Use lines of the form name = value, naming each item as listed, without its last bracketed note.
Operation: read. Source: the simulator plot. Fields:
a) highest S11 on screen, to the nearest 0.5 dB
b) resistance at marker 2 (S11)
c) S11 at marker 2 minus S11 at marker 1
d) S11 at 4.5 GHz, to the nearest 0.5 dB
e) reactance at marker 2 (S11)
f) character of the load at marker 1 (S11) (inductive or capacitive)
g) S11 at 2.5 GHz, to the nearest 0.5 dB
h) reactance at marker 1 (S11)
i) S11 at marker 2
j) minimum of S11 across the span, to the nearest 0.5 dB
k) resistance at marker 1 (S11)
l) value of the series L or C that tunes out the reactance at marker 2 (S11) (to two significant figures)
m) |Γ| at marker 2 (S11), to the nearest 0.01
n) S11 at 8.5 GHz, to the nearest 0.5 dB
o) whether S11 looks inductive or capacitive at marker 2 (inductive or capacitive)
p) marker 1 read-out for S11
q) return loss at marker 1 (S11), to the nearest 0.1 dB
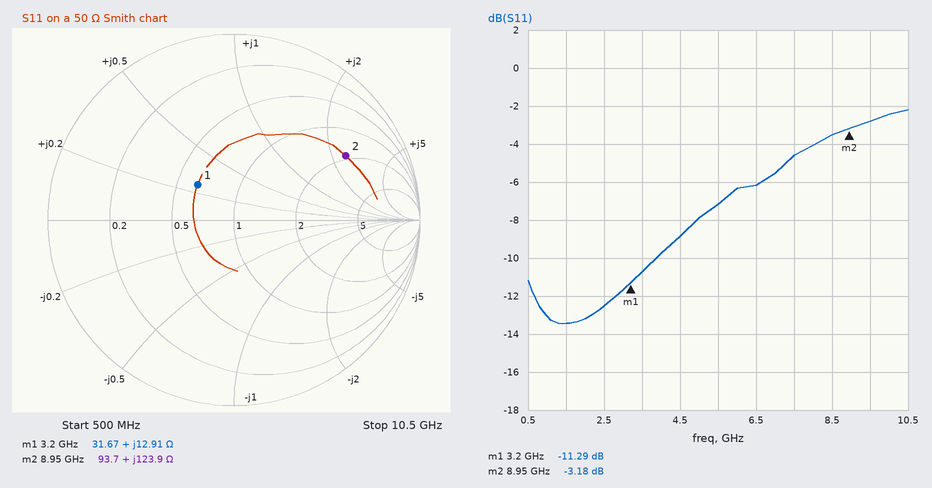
highest S11 on screen, to the nearest 0.5 dB = -2.0 dB
resistance at marker 2 = 93.7 Ω
S11 at marker 2 minus S11 at marker 1 = 8.11 dB
S11 at 4.5 GHz, to the nearest 0.5 dB = -9.0 dB
reactance at marker 2 = +123.9 Ω
character of the load at marker 1 (S11) = inductive
S11 at 2.5 GHz, to the nearest 0.5 dB = -12.5 dB
reactance at marker 1 = +12.91 Ω
S11 at marker 2 = -3.18 dB
minimum of S11 across the span, to the nearest 0.5 dB = -13.5 dB
resistance at marker 1 = 31.67 Ω
value of the series L or C that tunes out the reactance at marker 2 (S11) = 140 fF
|Γ| at marker 2 (S11), to the nearest 0.01 = 0.69
S11 at 8.5 GHz, to the nearest 0.5 dB = -3.5 dB
whether S11 looks inductive or capacitive at marker 2 = inductive
marker 1 read-out for S11 = -11.29 dB
return loss at marker 1 (S11), to the nearest 0.1 dB = 11.3 dB
